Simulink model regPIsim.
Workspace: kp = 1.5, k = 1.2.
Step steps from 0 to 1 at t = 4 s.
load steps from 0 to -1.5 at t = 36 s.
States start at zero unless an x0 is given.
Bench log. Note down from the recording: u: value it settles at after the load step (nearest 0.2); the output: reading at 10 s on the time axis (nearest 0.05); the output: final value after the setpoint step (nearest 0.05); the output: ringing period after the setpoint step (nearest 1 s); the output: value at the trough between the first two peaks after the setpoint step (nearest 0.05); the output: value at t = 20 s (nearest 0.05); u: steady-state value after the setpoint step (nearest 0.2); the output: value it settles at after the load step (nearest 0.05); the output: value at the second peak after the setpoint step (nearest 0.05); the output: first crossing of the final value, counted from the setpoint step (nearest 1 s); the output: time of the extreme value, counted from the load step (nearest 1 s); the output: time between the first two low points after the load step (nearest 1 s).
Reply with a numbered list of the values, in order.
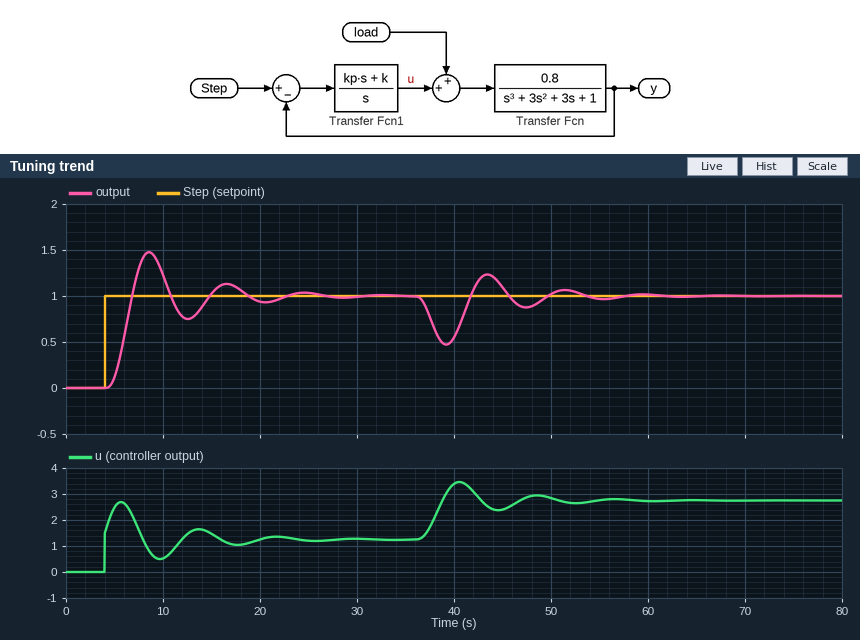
1. 2.8
2. 1.25
3. 1.00
4. 8 s
5. 0.75
6. 0.95
7. 1.2
8. 1.00
9. 1.15
10. 3 s
11. 3 s
12. 8 s
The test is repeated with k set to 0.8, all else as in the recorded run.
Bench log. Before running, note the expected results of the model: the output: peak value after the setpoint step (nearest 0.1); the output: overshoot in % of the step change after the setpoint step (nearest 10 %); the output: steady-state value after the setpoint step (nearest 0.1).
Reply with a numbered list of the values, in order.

1. 1.2
2. 20 %
3. 1.0
